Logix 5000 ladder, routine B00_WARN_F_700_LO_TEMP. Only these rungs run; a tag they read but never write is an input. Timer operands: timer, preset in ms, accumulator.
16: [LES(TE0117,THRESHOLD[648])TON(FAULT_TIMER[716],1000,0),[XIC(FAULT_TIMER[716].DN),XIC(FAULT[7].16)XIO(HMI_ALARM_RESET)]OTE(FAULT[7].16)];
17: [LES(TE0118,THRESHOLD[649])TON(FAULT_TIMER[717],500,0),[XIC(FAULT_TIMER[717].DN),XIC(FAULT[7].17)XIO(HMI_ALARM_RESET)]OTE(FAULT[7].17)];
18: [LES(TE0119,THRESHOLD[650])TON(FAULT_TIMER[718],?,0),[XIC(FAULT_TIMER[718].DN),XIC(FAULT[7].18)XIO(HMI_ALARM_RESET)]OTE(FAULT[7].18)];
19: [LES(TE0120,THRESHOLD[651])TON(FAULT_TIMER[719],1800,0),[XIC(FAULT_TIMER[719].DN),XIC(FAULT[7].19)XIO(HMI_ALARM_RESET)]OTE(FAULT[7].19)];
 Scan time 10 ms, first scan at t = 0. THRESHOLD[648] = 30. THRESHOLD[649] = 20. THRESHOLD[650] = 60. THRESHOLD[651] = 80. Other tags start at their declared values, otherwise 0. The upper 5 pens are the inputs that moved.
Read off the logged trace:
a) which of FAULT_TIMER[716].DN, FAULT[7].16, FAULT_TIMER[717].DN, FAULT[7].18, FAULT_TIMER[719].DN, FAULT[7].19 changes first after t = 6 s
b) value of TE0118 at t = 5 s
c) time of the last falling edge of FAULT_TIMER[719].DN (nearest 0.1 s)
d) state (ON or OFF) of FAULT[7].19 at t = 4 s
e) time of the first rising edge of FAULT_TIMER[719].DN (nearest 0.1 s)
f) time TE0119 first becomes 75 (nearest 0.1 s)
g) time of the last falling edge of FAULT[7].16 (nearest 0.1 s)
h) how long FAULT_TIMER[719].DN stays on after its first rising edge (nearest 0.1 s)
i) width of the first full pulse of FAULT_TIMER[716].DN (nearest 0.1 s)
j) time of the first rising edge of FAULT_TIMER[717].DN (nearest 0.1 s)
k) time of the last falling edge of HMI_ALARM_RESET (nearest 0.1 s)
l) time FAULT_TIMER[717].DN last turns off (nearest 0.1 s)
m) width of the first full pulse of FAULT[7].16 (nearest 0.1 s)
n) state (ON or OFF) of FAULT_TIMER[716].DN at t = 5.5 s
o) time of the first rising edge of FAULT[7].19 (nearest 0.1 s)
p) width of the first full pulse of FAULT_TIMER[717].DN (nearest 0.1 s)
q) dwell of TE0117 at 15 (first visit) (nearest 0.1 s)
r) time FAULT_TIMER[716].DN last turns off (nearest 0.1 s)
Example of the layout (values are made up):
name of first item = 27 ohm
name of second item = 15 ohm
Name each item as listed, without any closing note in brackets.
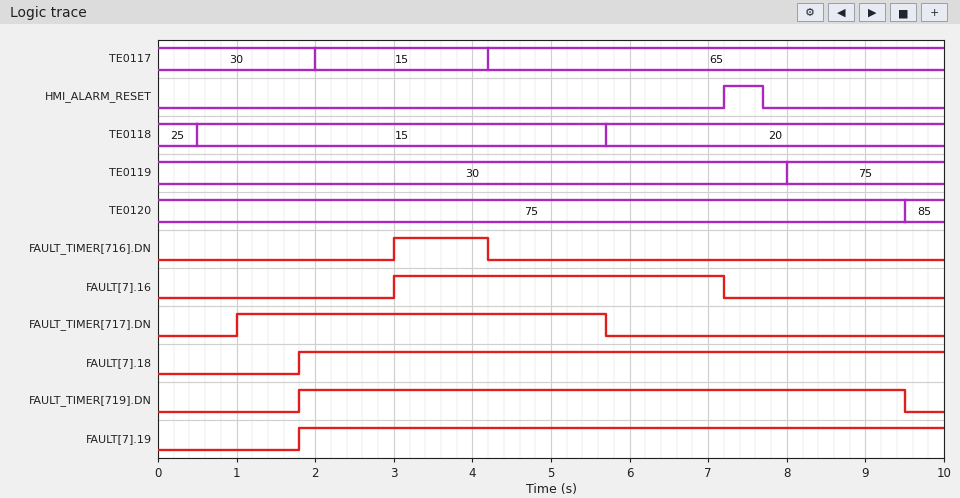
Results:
which of FAULT_TIMER[716].DN, FAULT[7].16, FAULT_TIMER[717].DN, FAULT[7].18, FAULT_TIMER[719].DN, FAULT[7].19 changes first after t = 6 s = FAULT[7].16
value of TE0118 at t = 5 s = 15
time of the last falling edge of FAULT_TIMER[719].DN = 9.5 s
state (ON or OFF) of FAULT[7].19 at t = 4 s = ON
time of the first rising edge of FAULT_TIMER[719].DN = 1.8 s
time TE0119 first becomes 75 = 8.0 s
time of the last falling edge of FAULT[7].16 = 7.2 s
how long FAULT_TIMER[719].DN stays on after its first rising edge = 7.7 s
width of the first full pulse of FAULT_TIMER[716].DN = 1.2 s
time of the first rising edge of FAULT_TIMER[717].DN = 1.0 s
time of the last falling edge of HMI_ALARM_RESET = 7.7 s
time FAULT_TIMER[717].DN last turns off = 5.7 s
width of the first full pulse of FAULT[7].16 = 4.2 s
state (ON or OFF) of FAULT_TIMER[716].DN at t = 5.5 s = OFF
time of the first rising edge of FAULT[7].19 = 1.8 s
width of the first full pulse of FAULT_TIMER[717].DN = 4.7 s
dwell of TE0117 at 15 (first visit) = 2.2 s
time FAULT_TIMER[716].DN last turns off = 4.2 s
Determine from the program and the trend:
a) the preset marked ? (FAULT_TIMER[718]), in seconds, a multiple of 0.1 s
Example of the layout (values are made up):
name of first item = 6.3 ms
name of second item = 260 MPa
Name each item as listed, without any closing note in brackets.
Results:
the preset marked ? (FAULT_TIMER[718]), in seconds, a multiple of 0.1 s = 1.8 s
